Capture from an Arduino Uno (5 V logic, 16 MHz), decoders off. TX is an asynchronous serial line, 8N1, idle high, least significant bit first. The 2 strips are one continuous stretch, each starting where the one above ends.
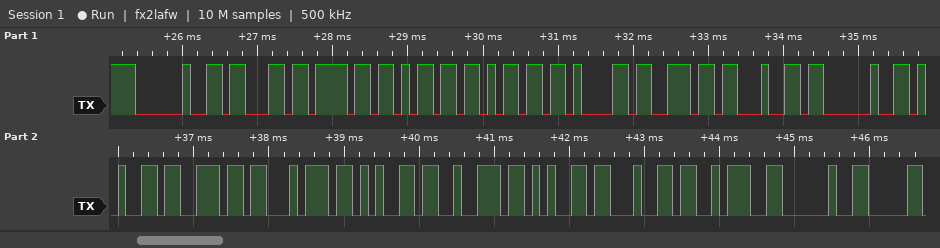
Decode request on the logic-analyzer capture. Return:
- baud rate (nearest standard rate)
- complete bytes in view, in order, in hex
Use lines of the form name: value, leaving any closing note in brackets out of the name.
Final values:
baud rate: 9600 baud
complete bytes in view, in order, in hex: 20 63 6F 6D 6D 61 6E 64 20 65 6E 74 65 72 65 64 3A 20
